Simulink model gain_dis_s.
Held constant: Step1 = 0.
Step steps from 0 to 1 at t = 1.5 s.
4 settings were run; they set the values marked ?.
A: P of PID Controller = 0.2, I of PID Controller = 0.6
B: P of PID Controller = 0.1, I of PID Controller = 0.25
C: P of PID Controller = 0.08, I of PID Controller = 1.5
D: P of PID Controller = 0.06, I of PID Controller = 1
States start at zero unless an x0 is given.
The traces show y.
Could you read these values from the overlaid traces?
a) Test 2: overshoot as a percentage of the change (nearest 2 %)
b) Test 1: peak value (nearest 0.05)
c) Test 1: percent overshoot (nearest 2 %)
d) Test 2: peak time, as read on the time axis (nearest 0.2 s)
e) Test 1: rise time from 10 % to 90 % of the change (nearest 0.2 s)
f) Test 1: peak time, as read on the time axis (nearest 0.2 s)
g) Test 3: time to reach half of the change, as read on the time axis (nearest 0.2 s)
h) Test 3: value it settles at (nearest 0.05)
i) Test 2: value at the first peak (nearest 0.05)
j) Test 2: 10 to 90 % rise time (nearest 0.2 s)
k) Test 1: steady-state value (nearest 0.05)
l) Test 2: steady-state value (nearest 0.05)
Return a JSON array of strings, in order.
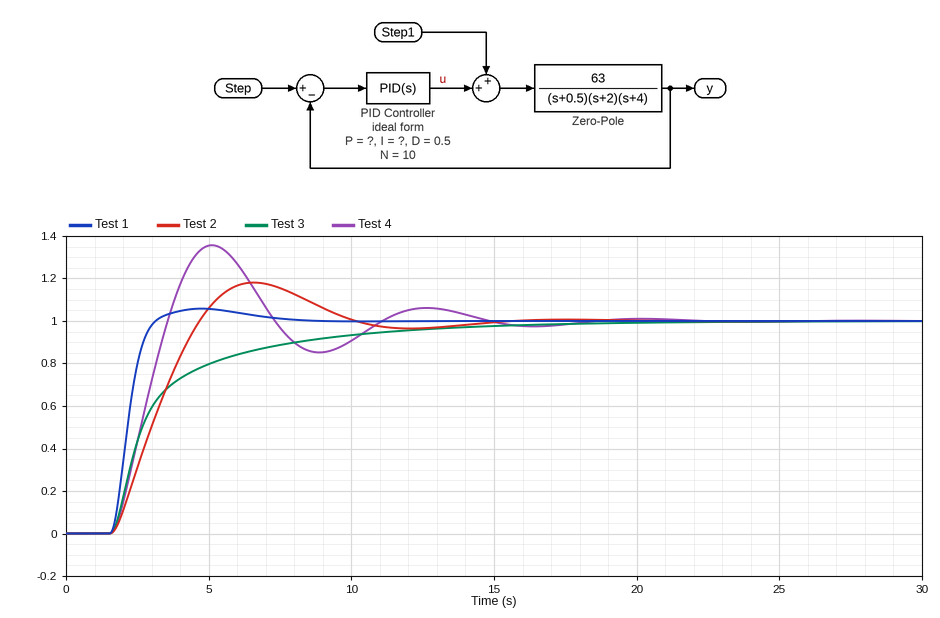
["18 %", "1.05", "6 %", "6.6 s", "1.0 s", "4.8 s", "2.6 s", "1.00", "1.20", "2.2 s", "1.00", "1.00"]
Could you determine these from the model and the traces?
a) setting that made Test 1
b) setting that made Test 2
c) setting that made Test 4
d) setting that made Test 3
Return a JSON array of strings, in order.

["A", "D", "C", "B"]
